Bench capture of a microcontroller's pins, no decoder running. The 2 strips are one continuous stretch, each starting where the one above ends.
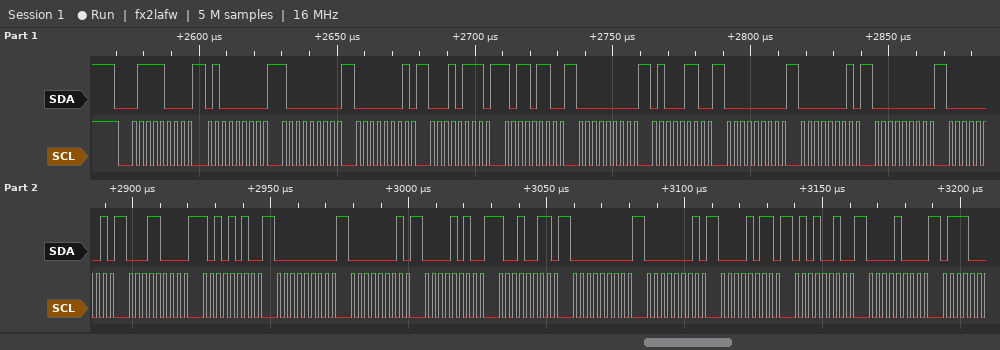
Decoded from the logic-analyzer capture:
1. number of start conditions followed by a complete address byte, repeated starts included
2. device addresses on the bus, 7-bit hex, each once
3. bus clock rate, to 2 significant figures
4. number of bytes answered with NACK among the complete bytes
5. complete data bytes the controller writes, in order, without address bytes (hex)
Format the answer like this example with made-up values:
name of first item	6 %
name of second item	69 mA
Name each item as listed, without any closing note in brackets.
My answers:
number of start conditions followed by a complete address byte, repeated starts included	1
device addresses on the bus, 7-bit hex, each once	0x3C
bus clock rate, to 2 significant figures	400 kHz
number of bytes answered with NACK among the complete bytes	0
complete data bytes the controller writes, in order, without address bytes	40 80 01 17 B6 00 46 00 01 00 01 18 AA 00 01 0A 93 00 01 0B 52 08
